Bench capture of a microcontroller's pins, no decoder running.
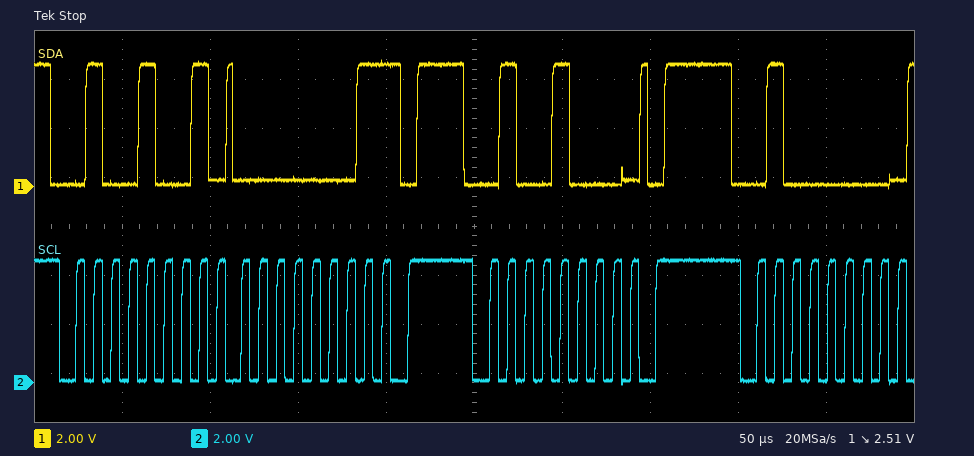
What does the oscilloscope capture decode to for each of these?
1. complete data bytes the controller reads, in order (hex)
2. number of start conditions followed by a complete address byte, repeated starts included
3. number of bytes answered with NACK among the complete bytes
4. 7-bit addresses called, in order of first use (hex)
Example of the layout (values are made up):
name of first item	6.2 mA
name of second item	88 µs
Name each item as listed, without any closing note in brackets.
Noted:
complete data bytes the controller reads, in order	01
number of start conditions followed by a complete address byte, repeated starts included	3
number of bytes answered with NACK among the complete bytes	1
7-bit addresses called, in order of first use	0x24 0x20
